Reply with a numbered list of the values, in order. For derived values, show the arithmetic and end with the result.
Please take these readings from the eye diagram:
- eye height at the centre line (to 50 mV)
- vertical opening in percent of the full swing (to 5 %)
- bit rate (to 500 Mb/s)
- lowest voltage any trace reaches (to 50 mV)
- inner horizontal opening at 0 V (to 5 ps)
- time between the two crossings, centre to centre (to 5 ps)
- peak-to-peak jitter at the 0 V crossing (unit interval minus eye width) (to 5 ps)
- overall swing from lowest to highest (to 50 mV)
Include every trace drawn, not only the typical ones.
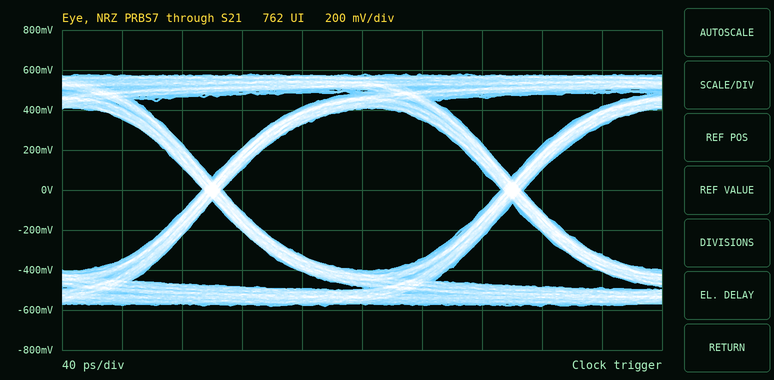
1. 800 mV
2. 800 mV / 1.15 V ≈ 70 %
3. 5.0 Gb/s
4. -600 mV
5. 185 ps
6. 200 ps
7. 15 ps
8. 1.15 V
